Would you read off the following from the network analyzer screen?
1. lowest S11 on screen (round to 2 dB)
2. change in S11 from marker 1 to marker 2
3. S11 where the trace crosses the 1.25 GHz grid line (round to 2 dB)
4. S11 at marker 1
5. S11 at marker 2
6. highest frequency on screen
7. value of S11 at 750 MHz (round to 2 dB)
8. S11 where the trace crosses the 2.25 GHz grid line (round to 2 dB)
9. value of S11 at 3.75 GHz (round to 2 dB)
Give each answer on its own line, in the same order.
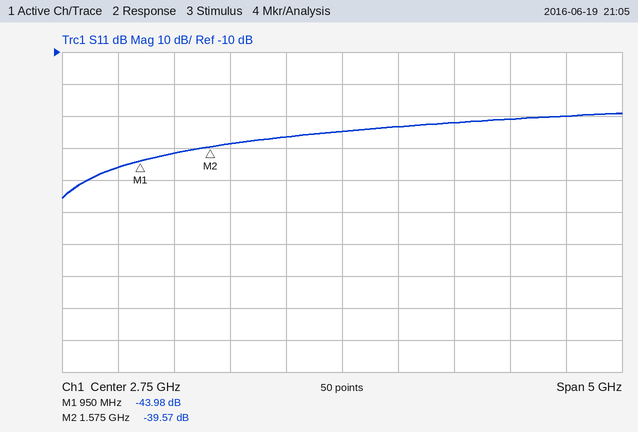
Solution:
-56 dB
4.41 dB
-42 dB
-43.98 dB
-39.57 dB
5.25 GHz
-46 dB
-36 dB
-32 dB
